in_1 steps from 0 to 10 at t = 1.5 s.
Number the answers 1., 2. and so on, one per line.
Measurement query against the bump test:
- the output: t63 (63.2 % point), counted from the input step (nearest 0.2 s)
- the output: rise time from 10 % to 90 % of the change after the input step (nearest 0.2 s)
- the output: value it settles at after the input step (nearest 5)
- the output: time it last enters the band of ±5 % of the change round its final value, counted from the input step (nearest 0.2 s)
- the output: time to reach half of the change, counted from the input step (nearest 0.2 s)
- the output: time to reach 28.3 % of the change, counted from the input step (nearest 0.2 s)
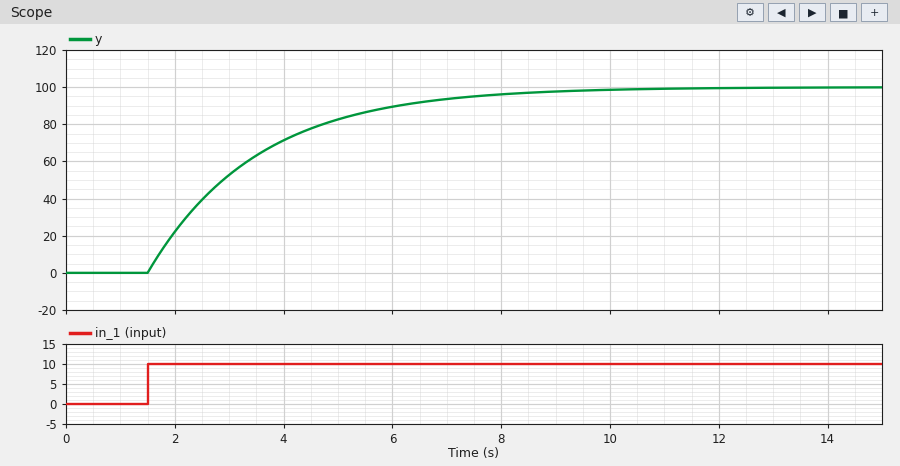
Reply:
1. 2.0 s
2. 4.4 s
3. 100
4. 6.0 s
5. 1.4 s
6. 0.6 s
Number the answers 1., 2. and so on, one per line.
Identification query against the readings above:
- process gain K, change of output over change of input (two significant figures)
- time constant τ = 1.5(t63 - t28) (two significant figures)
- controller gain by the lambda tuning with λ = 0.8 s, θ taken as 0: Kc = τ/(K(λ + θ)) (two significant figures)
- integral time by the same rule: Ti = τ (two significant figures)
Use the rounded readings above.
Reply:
1. 10
2. 2.1 s
3. 0.26
4. 2.1 s
